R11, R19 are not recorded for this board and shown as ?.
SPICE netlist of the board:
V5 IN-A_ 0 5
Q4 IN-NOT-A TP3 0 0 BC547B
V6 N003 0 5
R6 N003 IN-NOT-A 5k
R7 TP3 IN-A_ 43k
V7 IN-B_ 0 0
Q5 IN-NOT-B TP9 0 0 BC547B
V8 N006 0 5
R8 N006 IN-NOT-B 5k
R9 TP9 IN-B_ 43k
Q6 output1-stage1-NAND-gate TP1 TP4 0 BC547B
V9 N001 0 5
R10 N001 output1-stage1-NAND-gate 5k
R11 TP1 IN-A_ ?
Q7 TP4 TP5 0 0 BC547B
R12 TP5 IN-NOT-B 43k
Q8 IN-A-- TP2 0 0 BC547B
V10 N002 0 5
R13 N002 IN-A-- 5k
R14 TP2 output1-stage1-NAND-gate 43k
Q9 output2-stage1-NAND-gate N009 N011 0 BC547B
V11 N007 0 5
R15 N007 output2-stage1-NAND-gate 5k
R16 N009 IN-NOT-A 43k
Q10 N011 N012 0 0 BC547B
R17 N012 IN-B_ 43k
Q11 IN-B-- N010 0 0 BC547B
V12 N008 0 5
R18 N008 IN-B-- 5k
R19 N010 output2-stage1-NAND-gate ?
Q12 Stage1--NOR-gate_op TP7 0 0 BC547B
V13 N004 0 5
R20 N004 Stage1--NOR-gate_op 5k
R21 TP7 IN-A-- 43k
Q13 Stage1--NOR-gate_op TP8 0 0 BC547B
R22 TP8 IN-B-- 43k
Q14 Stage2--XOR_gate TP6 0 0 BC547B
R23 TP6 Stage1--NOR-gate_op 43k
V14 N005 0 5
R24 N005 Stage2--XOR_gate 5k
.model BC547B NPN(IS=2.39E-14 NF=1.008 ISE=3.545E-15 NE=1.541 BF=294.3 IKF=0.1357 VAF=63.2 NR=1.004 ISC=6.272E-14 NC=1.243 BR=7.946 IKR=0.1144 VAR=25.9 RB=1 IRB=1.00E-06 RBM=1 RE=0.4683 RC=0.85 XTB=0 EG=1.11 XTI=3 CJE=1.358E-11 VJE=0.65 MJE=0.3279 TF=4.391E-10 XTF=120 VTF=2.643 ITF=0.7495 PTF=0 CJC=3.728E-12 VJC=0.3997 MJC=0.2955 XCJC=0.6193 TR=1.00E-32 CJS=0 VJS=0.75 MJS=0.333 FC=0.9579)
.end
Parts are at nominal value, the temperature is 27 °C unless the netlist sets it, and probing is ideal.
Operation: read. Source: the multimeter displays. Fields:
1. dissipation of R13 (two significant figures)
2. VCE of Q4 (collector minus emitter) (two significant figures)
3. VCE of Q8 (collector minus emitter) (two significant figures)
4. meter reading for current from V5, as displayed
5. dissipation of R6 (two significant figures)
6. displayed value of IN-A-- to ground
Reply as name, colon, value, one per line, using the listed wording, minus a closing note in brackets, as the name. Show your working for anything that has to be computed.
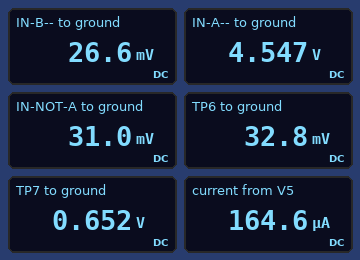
dissipation of R13: (5 V - 4.547 V)^2 / 5 kΩ = 41 µW
VCE of Q4 (collector minus emitter): 31 mV = 31 mV
VCE of Q8 (collector minus emitter): 4.547 V = 4.5 V
meter reading for current from V5, as displayed: 164.6 µA
dissipation of R6: (5 V - 31 mV)^2 / 5 kΩ = 4.9 mW
displayed value of IN-A-- to ground: 4.547 V
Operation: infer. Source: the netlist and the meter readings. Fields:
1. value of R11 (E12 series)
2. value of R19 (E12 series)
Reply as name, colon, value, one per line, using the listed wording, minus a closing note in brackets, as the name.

value of R11: 68 kΩ
value of R19: 27 kΩ
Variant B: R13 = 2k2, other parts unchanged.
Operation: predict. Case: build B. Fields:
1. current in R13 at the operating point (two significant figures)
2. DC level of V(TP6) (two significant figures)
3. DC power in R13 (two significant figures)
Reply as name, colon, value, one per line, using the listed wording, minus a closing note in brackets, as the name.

current in R13 at the operating point: 96 µA
DC level of V(TP6): 32 mV
DC power in R13: 20 µW
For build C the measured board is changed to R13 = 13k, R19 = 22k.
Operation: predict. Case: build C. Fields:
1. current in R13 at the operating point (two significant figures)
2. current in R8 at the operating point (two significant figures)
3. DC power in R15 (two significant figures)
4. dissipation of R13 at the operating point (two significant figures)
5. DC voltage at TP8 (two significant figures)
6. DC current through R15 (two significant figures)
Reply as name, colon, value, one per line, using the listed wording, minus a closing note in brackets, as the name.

current in R13 at the operating point: 78 µA
current in R8 at the operating point: 91 µA
DC power in R15: 130 µW
dissipation of R13 at the operating point: 78 µW
DC voltage at TP8: 24 mV
DC current through R15: 160 µA
